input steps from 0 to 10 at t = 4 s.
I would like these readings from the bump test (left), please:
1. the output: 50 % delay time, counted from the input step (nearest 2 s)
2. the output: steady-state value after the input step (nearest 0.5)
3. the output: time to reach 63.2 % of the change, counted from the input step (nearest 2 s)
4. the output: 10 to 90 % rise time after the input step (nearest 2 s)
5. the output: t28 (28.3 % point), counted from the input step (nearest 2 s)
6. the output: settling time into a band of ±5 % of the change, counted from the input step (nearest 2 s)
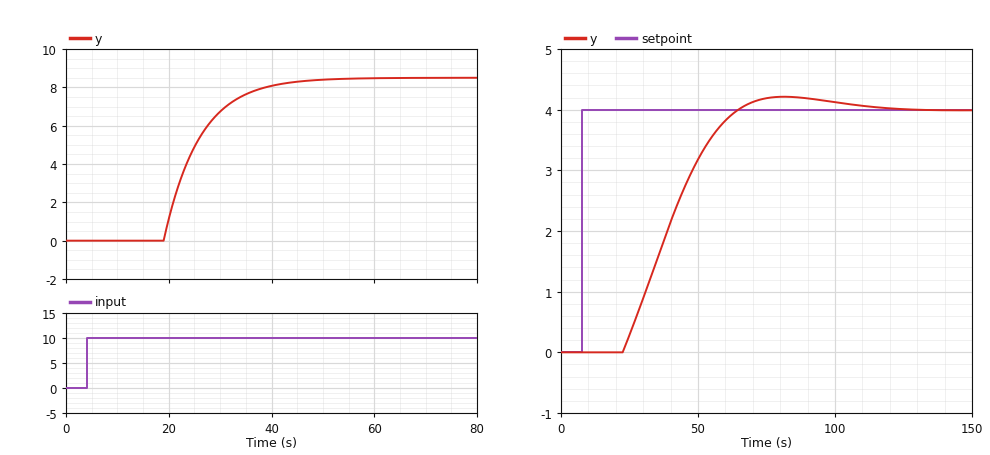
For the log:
20 s
8.5
22 s
16 s
18 s
36 s
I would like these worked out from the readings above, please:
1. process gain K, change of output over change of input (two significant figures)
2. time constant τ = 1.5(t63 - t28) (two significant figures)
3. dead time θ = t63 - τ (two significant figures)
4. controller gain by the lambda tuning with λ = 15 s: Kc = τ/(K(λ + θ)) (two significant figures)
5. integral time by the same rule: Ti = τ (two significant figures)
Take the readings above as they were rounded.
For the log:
0.85
6.0 s
16 s
0.23
6.0 s
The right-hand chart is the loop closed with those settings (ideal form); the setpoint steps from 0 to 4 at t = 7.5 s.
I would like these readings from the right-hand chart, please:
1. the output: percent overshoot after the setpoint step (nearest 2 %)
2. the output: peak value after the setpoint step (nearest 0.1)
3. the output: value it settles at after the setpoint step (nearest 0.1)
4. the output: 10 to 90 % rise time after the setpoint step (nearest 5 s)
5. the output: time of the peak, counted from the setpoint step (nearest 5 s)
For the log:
6 %
4.2
4.0
30 s
75 s
